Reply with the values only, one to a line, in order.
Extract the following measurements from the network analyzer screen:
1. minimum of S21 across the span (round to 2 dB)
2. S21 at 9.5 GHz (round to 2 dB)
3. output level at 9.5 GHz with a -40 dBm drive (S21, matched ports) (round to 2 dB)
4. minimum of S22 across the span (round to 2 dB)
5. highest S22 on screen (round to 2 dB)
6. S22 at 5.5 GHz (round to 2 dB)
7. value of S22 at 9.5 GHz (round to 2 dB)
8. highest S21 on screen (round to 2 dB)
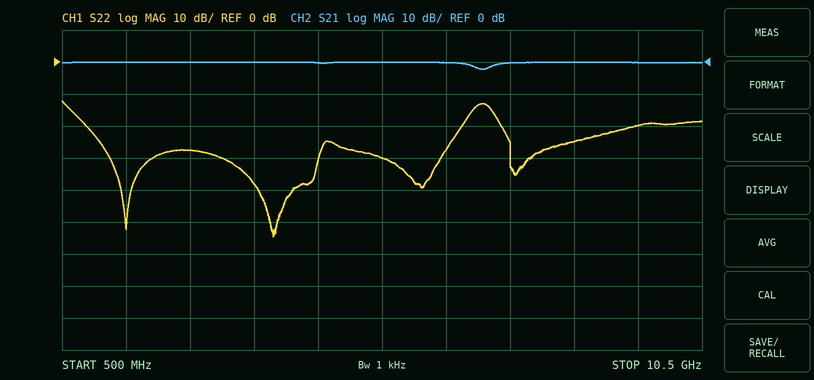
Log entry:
-2 dB
0 dB
-40 dBm
-54 dB
-12 dB
-30 dB
-20 dB
0 dB
